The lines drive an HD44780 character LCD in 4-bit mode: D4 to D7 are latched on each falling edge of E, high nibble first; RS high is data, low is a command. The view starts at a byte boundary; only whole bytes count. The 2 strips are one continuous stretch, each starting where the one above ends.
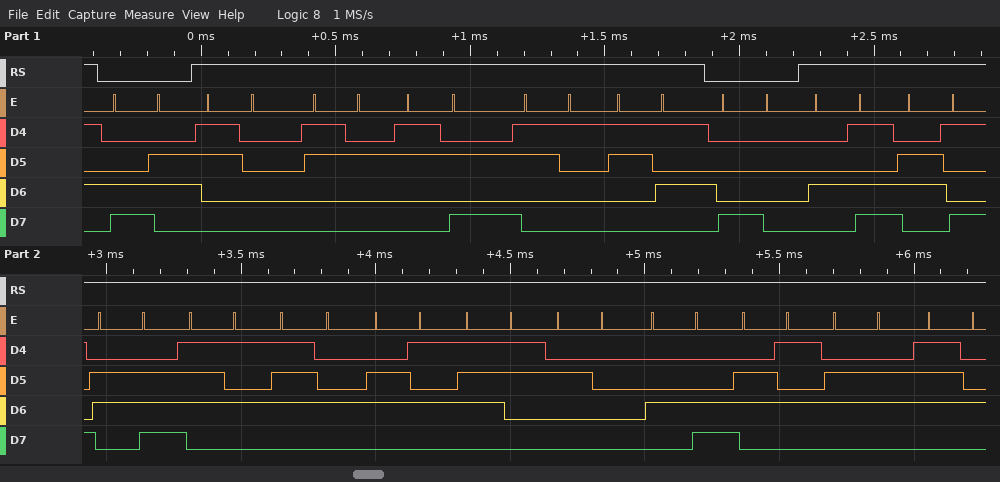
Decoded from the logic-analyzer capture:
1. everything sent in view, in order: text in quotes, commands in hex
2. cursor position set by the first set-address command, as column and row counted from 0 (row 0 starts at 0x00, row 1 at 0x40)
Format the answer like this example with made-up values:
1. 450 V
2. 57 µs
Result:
1. 0xC6 "02:15" 0x80 "Minutes Left"
2. column 6, row 1
